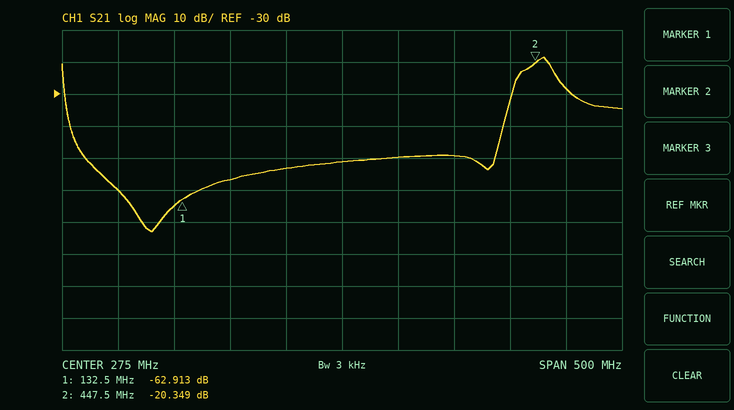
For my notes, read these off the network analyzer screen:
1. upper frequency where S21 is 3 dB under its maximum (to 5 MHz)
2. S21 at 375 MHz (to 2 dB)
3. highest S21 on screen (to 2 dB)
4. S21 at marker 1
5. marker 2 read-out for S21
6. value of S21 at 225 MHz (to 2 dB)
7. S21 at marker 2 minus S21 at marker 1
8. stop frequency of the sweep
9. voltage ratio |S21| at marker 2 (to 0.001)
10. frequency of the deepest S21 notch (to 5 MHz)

460 MHz
-50 dB
-18 dB
-62.913 dB
-20.349 dB
-54 dB
42.564 dB
525 MHz
0.096
105 MHz
